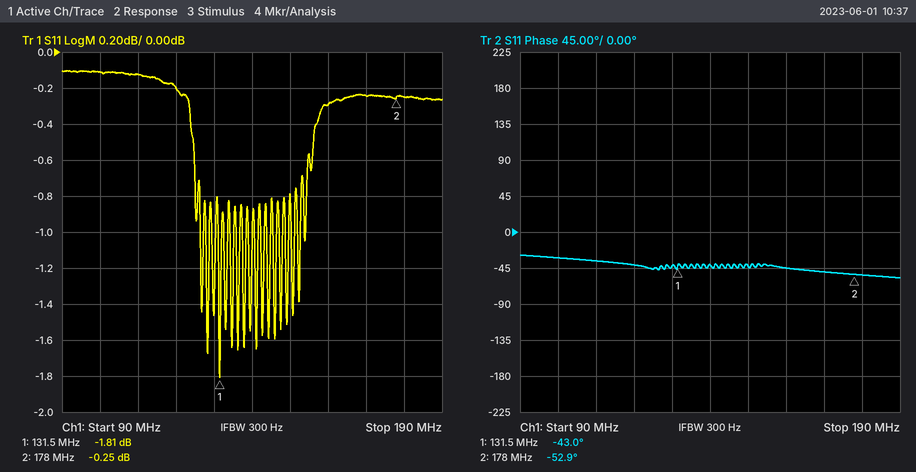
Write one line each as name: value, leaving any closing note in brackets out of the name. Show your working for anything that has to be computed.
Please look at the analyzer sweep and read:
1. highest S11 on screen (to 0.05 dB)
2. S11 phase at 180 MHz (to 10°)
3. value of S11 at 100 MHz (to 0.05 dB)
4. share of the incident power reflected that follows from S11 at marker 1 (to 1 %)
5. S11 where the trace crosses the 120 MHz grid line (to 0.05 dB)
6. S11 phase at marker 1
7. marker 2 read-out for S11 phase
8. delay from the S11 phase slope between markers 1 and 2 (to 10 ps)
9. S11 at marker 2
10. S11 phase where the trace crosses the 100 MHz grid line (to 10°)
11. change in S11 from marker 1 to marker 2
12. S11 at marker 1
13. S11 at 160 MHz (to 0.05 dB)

highest S11 on screen: -0.10 dB
S11 phase at 180 MHz: -50°
value of S11 at 100 MHz: -0.10 dB
share of the incident power reflected that follows from S11 at marker 1: 10^(-1.81/10) ≈ 66 %
S11 where the trace crosses the 120 MHz grid line: -0.20 dB
S11 phase at marker 1: -43.0°
marker 2 read-out for S11 phase: -52.9°
delay from the S11 phase slope between markers 1 and 2: −(-52.9° − (-43°))/(360° × 46.5 MHz) ≈ 591 ps, so 590 ps to the nearest 10 ps
S11 at marker 2: -0.25 dB
S11 phase where the trace crosses the 100 MHz grid line: -30°
change in S11 from marker 1 to marker 2: -0.25 − (-1.81) = 1.56 dB
S11 at marker 1: -1.81 dB
S11 at 160 MHz: -0.30 dB
